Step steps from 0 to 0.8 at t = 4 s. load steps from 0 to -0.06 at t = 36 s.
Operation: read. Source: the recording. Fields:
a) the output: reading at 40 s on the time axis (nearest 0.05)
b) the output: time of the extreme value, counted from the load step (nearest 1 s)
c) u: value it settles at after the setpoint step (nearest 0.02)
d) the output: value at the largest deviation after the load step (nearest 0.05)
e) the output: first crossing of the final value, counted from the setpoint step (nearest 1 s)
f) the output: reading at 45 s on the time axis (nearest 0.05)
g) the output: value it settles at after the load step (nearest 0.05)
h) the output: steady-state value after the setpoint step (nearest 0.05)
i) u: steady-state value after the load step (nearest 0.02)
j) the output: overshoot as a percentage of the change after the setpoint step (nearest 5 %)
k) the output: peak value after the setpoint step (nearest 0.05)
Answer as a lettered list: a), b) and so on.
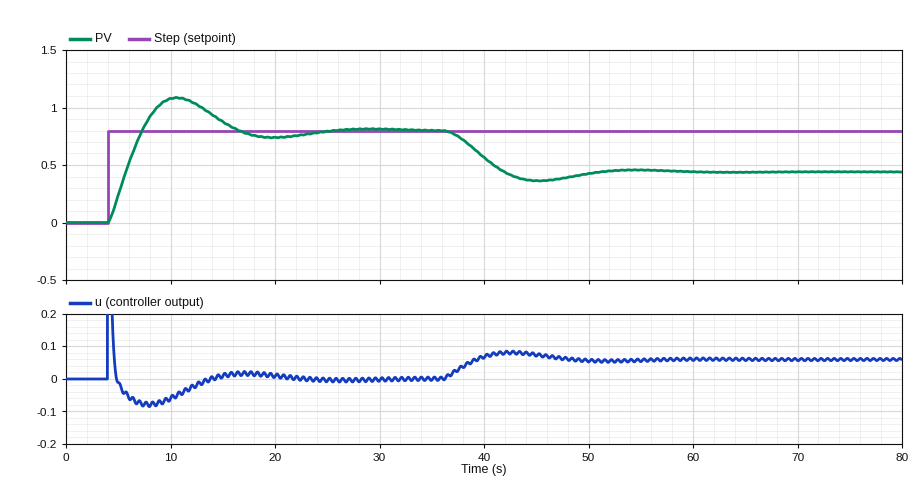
a) 0.55
b) 9 s
c) 0.00
d) 0.35
e) 3 s
f) 0.35
g) 0.45
h) 0.80
i) 0.06
j) 35 %
k) 1.10
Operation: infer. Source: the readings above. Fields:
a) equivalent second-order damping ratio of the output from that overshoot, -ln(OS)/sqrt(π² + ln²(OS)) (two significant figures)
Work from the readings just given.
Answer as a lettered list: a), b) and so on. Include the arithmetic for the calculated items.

a) ln(0.35) = -1.050; 1.050 / sqrt(9.870 + 1.102) = 0.32
